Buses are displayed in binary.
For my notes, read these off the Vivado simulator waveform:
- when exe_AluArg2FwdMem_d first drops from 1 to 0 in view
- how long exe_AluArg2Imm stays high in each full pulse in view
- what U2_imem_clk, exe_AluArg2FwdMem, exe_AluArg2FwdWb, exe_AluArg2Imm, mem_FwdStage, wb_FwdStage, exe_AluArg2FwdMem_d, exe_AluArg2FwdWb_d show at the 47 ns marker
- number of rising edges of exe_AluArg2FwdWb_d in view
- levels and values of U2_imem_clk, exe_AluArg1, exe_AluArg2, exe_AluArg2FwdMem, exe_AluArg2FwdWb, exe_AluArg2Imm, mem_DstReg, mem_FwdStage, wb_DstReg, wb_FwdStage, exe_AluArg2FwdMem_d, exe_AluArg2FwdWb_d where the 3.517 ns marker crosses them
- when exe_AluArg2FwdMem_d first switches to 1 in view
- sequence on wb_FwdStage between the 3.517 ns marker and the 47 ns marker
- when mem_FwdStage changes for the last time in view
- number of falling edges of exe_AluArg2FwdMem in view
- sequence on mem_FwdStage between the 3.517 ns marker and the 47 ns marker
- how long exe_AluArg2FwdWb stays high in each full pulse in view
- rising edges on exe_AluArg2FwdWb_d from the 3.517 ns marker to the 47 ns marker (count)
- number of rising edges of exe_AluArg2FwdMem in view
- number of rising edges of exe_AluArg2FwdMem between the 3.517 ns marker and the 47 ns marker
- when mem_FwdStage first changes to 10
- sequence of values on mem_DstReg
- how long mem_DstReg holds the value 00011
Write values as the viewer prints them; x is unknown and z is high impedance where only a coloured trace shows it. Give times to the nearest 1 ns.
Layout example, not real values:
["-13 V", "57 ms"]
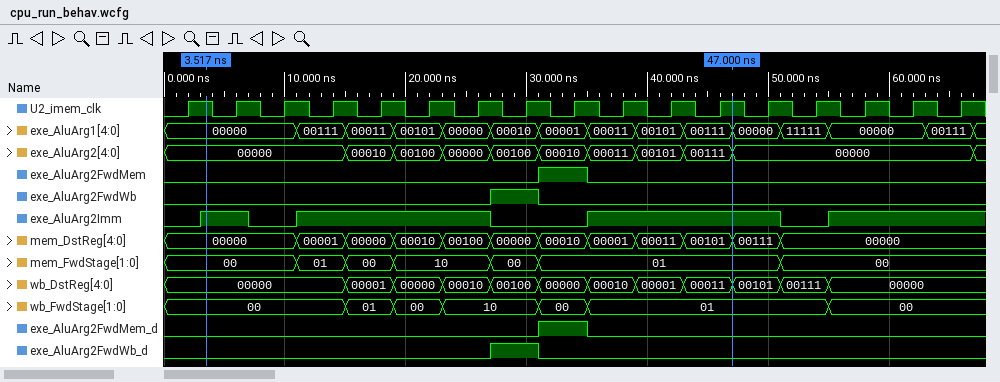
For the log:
["35 ns", "4 ns, 16 ns, 16 ns", "U2_imem_clk=1, exe_AluArg2FwdMem=0, exe_AluArg2FwdWb=0, exe_AluArg2Imm=1, mem_FwdStage=01, wb_FwdStage=01, exe_AluArg2FwdMem_d=0, exe_AluArg2FwdWb_d=0", "1", "U2_imem_clk=1, exe_AluArg1=00000, exe_AluArg2=00000, exe_AluArg2FwdMem=0, exe_AluArg2FwdWb=0, exe_AluArg2Imm=1, mem_DstReg=00000, mem_FwdStage=00, wb_DstReg=00000, wb_FwdStage=00, exe_AluArg2FwdMem_d=0, exe_AluArg2FwdWb_d=0", "31 ns", "00, 01, 00, 10, 00, 01", "51 ns", "1", "00, 01, 00, 10, 00, 01", "4 ns", "1", "1", "1", "19 ns", "00000, 00001, 00000, 00010, 00100, 00000, 00010, 00001, 00011, 00101, 00111, 00000", "4 ns"]
